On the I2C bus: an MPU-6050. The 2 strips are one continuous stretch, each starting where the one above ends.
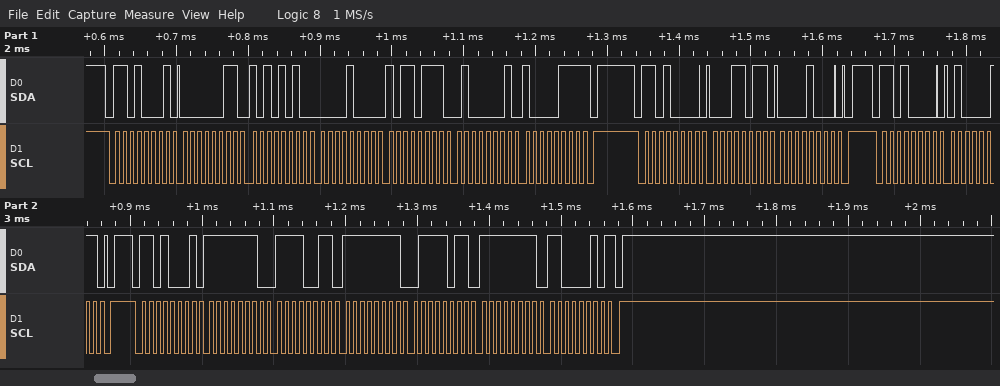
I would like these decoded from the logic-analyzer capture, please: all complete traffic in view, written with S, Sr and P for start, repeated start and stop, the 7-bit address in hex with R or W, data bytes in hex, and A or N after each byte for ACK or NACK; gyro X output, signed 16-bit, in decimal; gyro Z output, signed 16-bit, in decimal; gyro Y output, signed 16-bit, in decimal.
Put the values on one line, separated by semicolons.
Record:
S 68R A 03 A AA A 08 A B7 A 41 A 87 N P S 68W A 1B A 08 A P S 68W A 43 A P S 68R A FE A F3 A FF A 7B A FF A C2 N P; -269; -62; -133
